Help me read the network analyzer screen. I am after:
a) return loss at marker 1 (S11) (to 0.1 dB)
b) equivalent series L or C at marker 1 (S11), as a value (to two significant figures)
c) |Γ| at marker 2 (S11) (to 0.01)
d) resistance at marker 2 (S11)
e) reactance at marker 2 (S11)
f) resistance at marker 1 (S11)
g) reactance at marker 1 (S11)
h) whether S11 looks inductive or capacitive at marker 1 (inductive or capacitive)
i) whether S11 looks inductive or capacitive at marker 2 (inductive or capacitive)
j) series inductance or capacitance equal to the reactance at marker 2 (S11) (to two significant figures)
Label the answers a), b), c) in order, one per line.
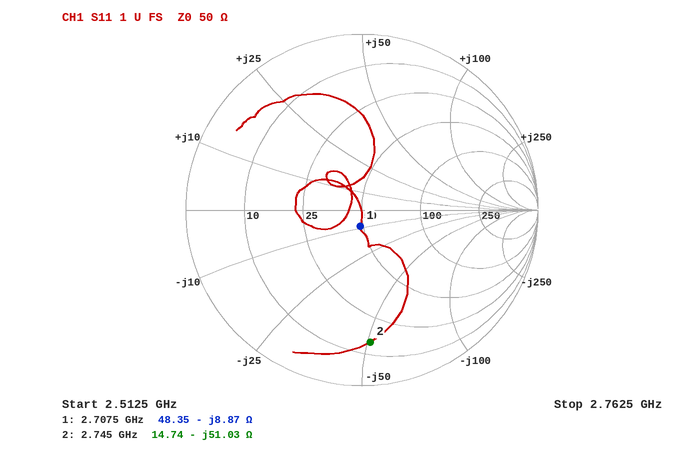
a) 20.8 dB
b) 6.6 pF
c) 0.75
d) 14.74 Ω
e) -51.03 Ω
f) 48.35 Ω
g) -8.87 Ω
h) capacitive
i) capacitive
j) 1.1 pF
